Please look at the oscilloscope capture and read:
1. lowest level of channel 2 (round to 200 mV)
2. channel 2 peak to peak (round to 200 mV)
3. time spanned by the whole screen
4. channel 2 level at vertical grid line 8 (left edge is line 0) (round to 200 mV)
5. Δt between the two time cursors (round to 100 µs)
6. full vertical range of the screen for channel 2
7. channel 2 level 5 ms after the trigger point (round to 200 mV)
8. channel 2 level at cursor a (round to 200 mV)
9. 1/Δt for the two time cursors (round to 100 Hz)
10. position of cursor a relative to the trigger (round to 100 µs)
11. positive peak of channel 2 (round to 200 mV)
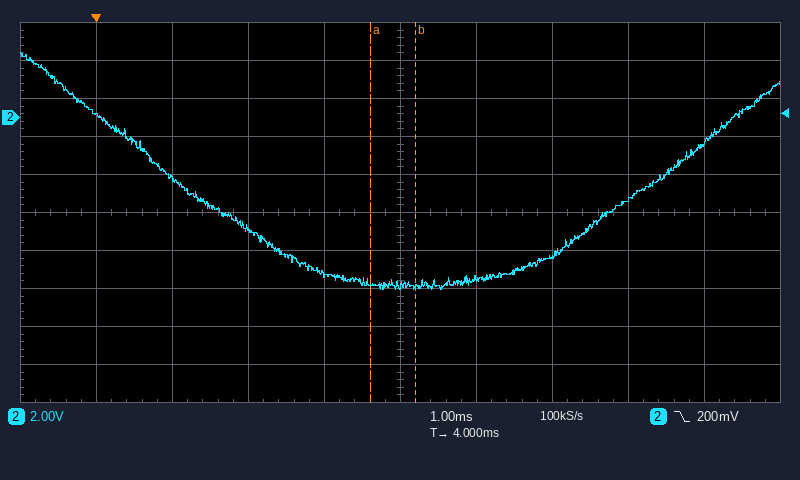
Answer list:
-9.0 V
12.4 V
10 ms
-4.4 V
600 µs
20 V
-8.4 V
-8.6 V
1.7 kHz
+3.6 ms
3.4 V
